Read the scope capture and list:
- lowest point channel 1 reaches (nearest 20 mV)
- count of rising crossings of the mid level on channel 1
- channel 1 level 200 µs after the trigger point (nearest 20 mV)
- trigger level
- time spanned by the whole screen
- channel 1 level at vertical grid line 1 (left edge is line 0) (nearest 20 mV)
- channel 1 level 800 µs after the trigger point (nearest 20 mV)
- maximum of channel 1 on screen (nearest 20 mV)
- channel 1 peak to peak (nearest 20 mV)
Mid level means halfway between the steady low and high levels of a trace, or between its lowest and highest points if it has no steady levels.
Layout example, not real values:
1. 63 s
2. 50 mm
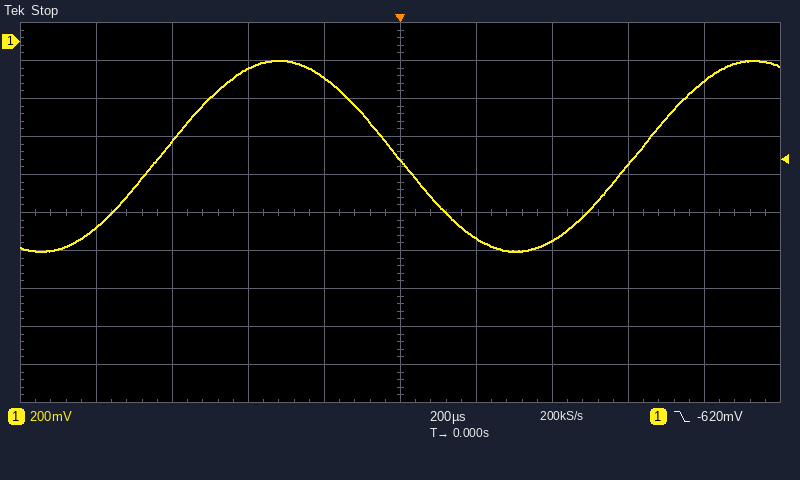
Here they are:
1. -1.10 V
2. 2
3. -1.04 V
4. -620 mV
5. 2 ms
6. -980 mV
7. -200 mV
8. -100 mV
9. 1.00 V
